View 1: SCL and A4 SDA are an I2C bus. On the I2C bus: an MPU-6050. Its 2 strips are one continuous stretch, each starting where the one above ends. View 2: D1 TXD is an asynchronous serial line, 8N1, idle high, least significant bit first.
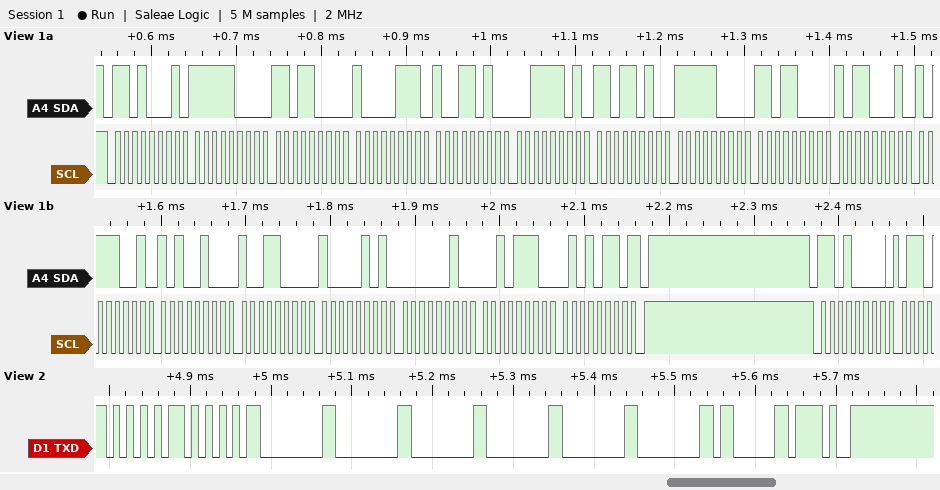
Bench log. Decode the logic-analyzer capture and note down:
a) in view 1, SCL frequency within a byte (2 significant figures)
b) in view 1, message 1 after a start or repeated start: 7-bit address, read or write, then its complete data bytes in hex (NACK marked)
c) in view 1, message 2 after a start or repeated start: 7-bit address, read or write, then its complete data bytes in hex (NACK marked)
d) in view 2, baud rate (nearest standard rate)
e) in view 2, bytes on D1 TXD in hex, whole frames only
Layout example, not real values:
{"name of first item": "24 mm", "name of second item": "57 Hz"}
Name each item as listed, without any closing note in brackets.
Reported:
{"in view 1, SCL frequency within a byte": "100 kHz", "in view 1, message 1 after a start or repeated start: 7-bit address, read or write, then its complete data bytes in hex": "0x68 read: F8 D8 87 9A 3D DA F8 D8 B1 B9 A4 98 85 02 2E 56 NACK", "in view 1, message 2 after a start or repeated start: 7-bit address, read or write, then its complete data bytes in hex": "0x68 write", "in view 2, baud rate": "115200 baud", "in view 2, bytes on D1 TXD in hex, whole frames only": "55 55 00 00 00 00 00 00 03 2F"}
